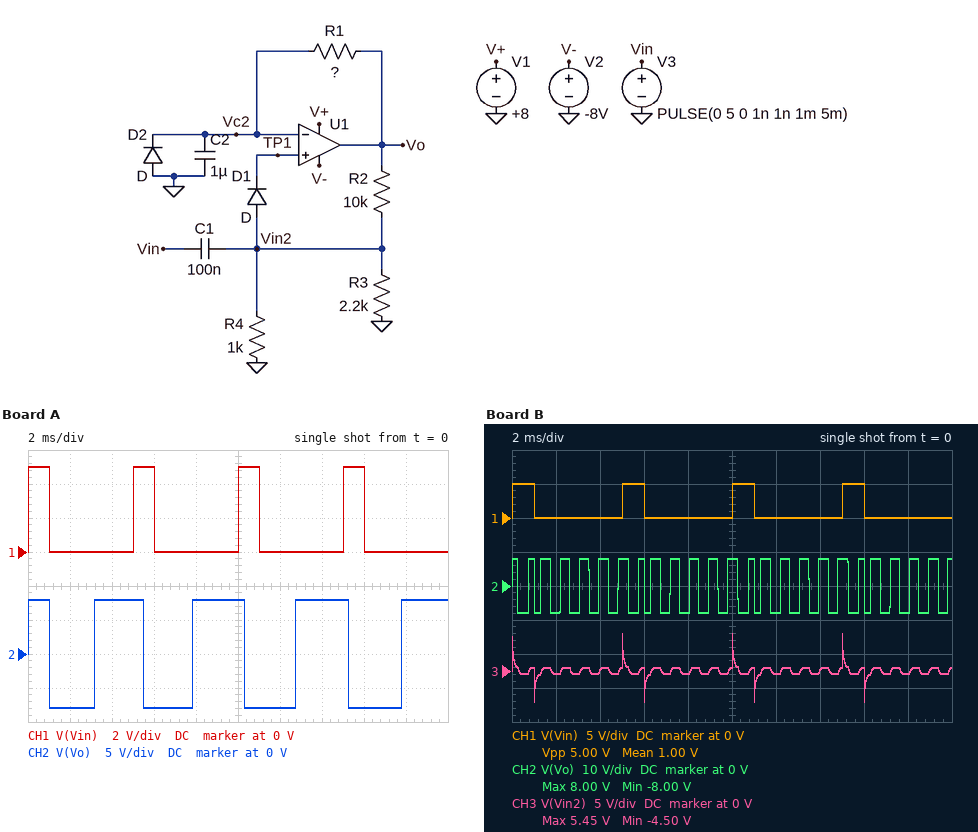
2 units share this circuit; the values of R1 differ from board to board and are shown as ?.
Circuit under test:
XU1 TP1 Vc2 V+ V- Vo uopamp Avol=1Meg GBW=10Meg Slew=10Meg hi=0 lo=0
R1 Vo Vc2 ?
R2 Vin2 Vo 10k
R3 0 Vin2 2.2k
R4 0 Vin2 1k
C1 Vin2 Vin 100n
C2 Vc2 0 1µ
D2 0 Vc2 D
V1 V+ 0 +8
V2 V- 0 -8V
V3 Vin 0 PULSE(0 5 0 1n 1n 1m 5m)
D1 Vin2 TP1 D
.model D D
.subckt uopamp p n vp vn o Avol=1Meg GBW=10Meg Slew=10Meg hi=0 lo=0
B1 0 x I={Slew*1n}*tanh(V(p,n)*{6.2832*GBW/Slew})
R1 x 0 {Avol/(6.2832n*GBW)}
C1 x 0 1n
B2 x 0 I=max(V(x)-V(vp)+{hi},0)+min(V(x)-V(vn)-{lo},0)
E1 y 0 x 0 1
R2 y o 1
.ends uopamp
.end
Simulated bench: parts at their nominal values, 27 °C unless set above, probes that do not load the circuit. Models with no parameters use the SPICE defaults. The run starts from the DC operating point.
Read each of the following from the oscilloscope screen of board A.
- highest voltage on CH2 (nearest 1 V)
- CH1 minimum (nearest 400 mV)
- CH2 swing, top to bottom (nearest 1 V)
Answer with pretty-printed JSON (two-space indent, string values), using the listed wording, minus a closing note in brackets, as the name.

{
  "highest voltage on CH2": "8 V",
  "CH1 minimum": "0 V",
  "CH2 swing, top to bottom": "16 V"
}
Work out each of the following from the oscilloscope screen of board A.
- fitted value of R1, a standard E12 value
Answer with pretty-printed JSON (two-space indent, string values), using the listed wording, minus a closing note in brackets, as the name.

{
  "fitted value of R1, a standard E12 value": "18 kΩ"
}
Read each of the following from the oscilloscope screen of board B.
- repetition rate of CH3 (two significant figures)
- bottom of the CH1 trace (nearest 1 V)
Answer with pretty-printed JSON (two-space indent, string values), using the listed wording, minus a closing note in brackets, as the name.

{
  "repetition rate of CH3": "200 Hz",
  "bottom of the CH1 trace": "0 V"
}
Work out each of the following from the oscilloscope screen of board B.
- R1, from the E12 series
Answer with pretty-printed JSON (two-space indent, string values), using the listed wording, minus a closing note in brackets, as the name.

{
  "R1, from the E12 series": "3.3 kΩ"
}
